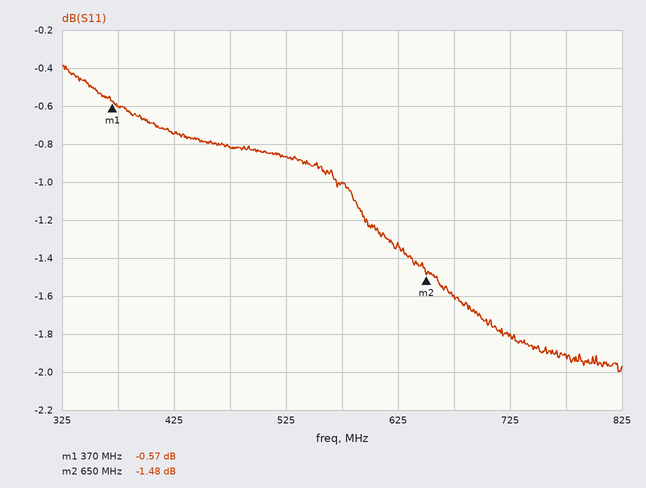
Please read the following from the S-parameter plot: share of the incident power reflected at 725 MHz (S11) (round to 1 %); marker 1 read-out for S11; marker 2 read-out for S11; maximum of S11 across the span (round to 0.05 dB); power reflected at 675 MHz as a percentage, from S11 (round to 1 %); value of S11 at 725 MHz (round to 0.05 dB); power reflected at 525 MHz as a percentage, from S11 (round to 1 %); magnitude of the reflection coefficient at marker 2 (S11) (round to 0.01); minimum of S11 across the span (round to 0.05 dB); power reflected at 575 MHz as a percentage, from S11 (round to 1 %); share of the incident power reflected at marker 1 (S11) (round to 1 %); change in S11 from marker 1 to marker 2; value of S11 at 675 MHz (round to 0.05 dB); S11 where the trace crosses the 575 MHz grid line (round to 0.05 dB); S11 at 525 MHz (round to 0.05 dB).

66 %
-0.57 dB
-1.48 dB
-0.40 dB
69 %
-1.80 dB
82 %
0.84
-2.00 dB
79 %
88 %
-0.91 dB
-1.60 dB
-1.00 dB
-0.85 dB
